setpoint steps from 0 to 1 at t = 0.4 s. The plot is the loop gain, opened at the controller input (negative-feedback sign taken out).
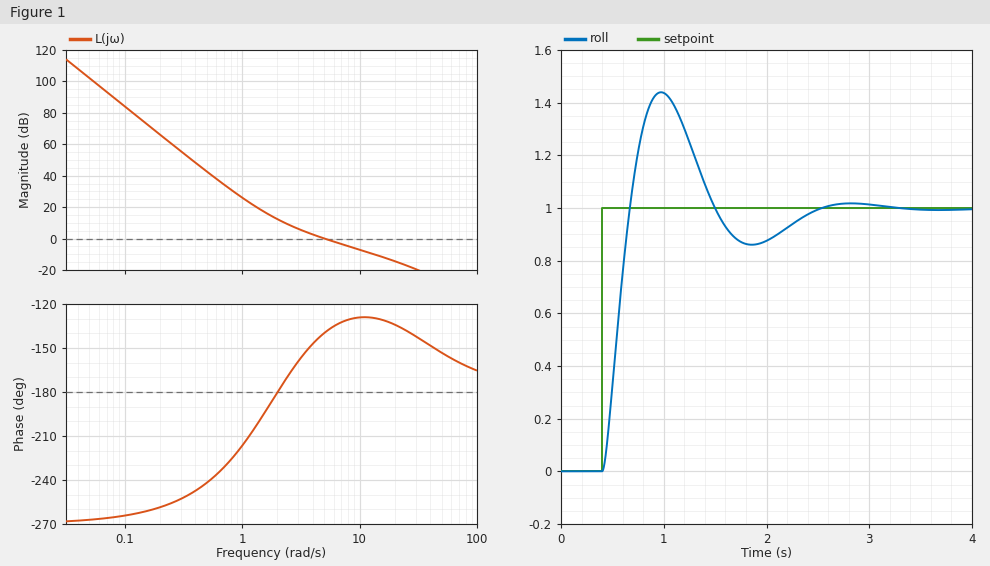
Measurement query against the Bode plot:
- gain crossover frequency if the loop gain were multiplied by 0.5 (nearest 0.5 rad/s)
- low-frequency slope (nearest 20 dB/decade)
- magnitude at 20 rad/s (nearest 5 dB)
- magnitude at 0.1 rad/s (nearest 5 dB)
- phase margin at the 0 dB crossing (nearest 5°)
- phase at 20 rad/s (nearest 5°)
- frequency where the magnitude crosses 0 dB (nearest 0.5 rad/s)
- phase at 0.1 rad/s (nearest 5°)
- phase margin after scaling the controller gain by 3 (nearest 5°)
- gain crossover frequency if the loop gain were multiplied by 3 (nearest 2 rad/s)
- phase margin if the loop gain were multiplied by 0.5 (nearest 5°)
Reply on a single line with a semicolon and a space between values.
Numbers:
3.0 rad/s; -60 dB/decade; -15 dB; 85 dB; 40°; -135°; 5.0 rad/s; -265°; 50°; 12 rad/s; 20°
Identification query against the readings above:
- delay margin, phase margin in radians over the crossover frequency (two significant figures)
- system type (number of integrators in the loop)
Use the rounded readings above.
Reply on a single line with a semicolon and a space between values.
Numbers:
0.14 s; 3
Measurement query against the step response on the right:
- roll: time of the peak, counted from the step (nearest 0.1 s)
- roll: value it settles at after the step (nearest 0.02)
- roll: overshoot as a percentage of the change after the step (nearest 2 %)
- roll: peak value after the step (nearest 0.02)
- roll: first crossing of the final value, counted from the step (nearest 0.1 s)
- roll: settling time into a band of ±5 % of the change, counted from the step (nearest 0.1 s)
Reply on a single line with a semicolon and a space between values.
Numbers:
0.6 s; 1.00; 44 %; 1.44; 0.3 s; 1.9 s
